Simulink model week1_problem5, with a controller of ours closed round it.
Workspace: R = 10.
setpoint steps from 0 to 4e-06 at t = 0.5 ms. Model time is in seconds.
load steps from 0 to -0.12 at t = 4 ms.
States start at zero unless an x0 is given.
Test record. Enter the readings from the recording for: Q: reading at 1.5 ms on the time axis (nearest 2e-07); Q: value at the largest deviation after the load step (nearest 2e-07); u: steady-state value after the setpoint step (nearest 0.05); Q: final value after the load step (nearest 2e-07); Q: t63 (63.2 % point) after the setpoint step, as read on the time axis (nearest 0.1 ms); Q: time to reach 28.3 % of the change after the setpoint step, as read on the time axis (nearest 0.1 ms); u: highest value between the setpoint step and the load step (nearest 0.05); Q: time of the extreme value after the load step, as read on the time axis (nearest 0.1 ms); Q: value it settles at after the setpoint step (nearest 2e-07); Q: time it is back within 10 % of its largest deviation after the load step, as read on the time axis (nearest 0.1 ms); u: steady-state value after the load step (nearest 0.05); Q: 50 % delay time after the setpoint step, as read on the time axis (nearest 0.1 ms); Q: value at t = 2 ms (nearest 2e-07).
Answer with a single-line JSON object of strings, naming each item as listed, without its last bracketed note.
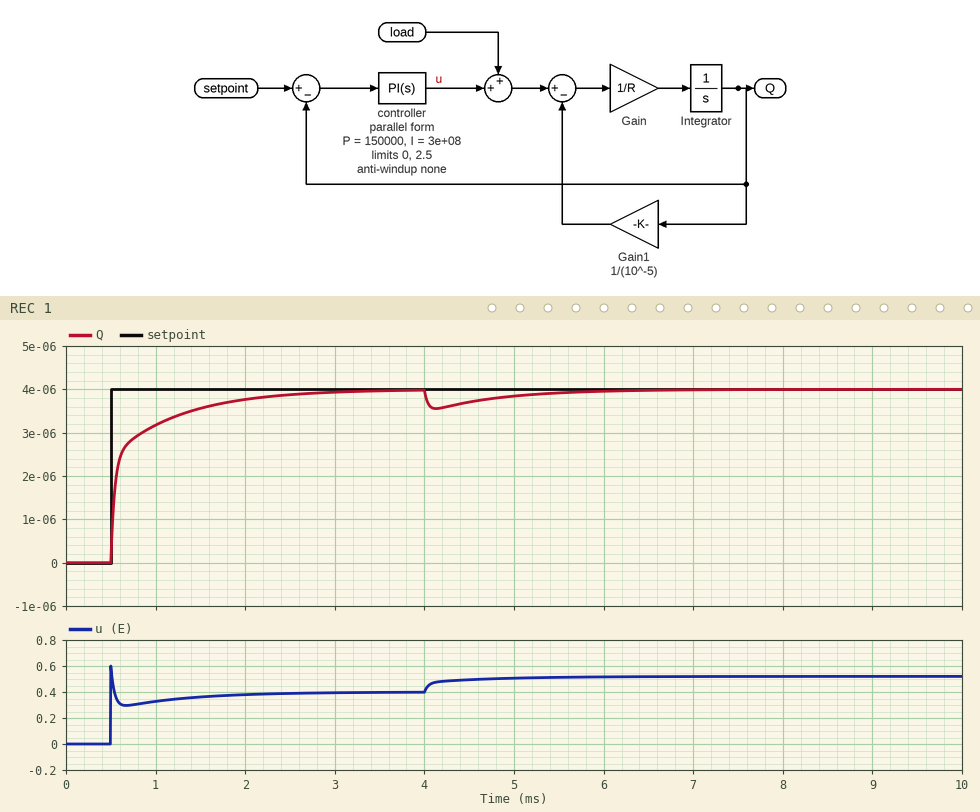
{"Q: reading at 1.5 ms on the time axis": "0.0000036", "Q: value at the largest deviation after the load step": "0.0000036", "u: steady-state value after the setpoint step": "0.40", "Q: final value after the load step": "0.0000040", "Q: t63 (63.2 % point) after the setpoint step, as read on the time axis": "0.6 ms", "Q: time to reach 28.3 % of the change after the setpoint step, as read on the time axis": "0.5 ms", "u: highest value between the setpoint step and the load step": "0.60", "Q: time of the extreme value after the load step, as read on the time axis": "4.1 ms", "Q: value it settles at after the setpoint step": "0.0000040", "Q: time it is back within 10 % of its largest deviation after the load step, as read on the time axis": "6.0 ms", "u: steady-state value after the load step": "0.50", "Q: 50 % delay time after the setpoint step, as read on the time axis": "0.6 ms", "Q: value at t = 2 ms": "0.0000038"}
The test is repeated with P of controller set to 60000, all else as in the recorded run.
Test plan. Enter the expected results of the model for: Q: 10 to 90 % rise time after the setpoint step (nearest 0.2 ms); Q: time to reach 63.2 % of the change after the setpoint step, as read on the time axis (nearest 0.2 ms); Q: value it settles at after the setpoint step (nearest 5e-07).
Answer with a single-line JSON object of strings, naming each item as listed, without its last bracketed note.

{"Q: 10 to 90 % rise time after the setpoint step": "0.8 ms", "Q: time to reach 63.2 % of the change after the setpoint step, as read on the time axis": "0.8 ms", "Q: value it settles at after the setpoint step": "0.0000040"}
